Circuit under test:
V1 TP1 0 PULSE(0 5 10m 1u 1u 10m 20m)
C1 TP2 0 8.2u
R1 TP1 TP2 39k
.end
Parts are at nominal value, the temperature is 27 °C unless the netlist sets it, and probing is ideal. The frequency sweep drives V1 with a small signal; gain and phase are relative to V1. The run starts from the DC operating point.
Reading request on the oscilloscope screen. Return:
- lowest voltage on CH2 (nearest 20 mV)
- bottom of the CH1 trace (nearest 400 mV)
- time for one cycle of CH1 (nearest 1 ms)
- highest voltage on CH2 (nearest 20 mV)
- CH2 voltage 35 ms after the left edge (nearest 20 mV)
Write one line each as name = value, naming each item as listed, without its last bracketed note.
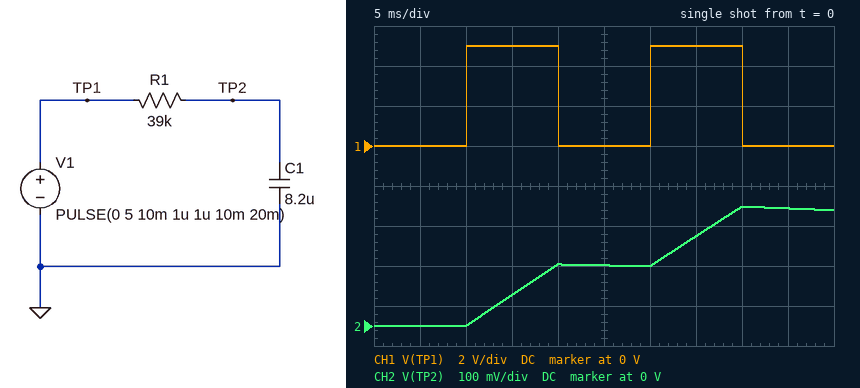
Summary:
lowest voltage on CH2 = 0 V
bottom of the CH1 trace = 0 V
time for one cycle of CH1 = 20 ms
highest voltage on CH2 = 300 mV
CH2 voltage 35 ms after the left edge = 220 mV
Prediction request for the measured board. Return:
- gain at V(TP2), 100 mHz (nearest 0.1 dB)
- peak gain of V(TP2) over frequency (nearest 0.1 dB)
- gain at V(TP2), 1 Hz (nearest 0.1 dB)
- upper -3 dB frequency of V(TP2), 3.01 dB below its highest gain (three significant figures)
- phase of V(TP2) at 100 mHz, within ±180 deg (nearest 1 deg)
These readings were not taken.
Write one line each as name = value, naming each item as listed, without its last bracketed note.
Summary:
gain at V(TP2), 100 mHz = -0.2 dB
peak gain of V(TP2) over frequency = 0 dB
gain at V(TP2), 1 Hz = -7.0 dB
upper -3 dB frequency of V(TP2), 3.01 dB below its highest gain = 498 mHz
phase of V(TP2) at 100 mHz, within ±180 deg = -11 deg
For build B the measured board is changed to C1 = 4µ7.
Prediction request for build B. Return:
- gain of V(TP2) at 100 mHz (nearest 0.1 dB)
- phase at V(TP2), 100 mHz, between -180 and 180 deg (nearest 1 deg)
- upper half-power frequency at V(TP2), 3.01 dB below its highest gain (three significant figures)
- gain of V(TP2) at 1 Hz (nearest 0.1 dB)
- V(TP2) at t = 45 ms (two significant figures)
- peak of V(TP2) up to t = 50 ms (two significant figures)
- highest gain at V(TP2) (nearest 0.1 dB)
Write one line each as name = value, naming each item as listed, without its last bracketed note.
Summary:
gain of V(TP2) at 100 mHz = -0.1 dB
phase at V(TP2), 100 mHz, between -180 and 180 deg = -7 deg
upper half-power frequency at V(TP2), 3.01 dB below its highest gain = 868 mHz
gain of V(TP2) at 1 Hz = -3.7 dB
V(TP2) at t = 45 ms = 490 mV
peak of V(TP2) up to t = 50 ms = 500 mV
highest gain at V(TP2) = 0 dB
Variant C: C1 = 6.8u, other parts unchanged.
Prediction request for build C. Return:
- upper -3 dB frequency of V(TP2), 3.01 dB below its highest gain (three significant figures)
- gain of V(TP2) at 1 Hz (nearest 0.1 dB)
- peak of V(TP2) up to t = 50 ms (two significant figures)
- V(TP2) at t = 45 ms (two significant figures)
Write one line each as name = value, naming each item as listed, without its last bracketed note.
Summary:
upper -3 dB frequency of V(TP2), 3.01 dB below its highest gain = 600 mHz
gain of V(TP2) at 1 Hz = -5.8 dB
peak of V(TP2) up to t = 50 ms = 360 mV
V(TP2) at t = 45 ms = 350 mV
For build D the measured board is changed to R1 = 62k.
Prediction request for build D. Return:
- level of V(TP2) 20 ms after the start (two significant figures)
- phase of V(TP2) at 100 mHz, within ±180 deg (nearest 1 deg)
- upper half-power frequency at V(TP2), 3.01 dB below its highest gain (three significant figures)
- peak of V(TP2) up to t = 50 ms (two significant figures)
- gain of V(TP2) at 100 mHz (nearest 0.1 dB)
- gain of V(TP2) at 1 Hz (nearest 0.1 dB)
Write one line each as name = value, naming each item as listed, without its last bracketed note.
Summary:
level of V(TP2) 20 ms after the start = 97 mV
phase of V(TP2) at 100 mHz, within ±180 deg = -18 deg
upper half-power frequency at V(TP2), 3.01 dB below its highest gain = 313 mHz
peak of V(TP2) up to t = 50 ms = 190 mV
gain of V(TP2) at 100 mHz = -0.4 dB
gain of V(TP2) at 1 Hz = -10.5 dB
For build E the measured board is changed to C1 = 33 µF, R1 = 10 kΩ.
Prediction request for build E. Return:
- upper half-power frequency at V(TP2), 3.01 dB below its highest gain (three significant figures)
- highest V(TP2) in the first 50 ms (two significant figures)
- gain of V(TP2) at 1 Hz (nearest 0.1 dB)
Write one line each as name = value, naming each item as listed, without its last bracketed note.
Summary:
upper half-power frequency at V(TP2), 3.01 dB below its highest gain = 482 mHz
highest V(TP2) in the first 50 ms = 290 mV
gain of V(TP2) at 1 Hz = -7.2 dB
